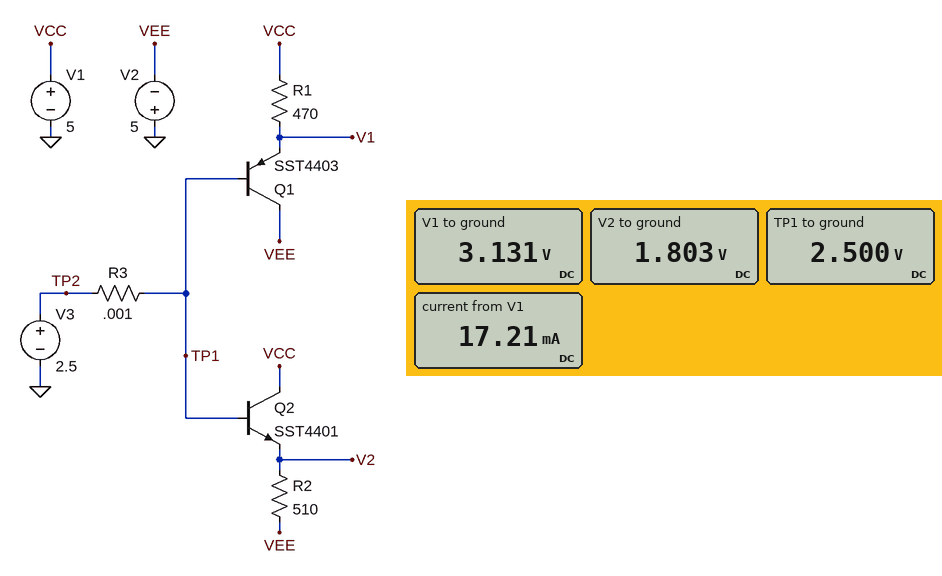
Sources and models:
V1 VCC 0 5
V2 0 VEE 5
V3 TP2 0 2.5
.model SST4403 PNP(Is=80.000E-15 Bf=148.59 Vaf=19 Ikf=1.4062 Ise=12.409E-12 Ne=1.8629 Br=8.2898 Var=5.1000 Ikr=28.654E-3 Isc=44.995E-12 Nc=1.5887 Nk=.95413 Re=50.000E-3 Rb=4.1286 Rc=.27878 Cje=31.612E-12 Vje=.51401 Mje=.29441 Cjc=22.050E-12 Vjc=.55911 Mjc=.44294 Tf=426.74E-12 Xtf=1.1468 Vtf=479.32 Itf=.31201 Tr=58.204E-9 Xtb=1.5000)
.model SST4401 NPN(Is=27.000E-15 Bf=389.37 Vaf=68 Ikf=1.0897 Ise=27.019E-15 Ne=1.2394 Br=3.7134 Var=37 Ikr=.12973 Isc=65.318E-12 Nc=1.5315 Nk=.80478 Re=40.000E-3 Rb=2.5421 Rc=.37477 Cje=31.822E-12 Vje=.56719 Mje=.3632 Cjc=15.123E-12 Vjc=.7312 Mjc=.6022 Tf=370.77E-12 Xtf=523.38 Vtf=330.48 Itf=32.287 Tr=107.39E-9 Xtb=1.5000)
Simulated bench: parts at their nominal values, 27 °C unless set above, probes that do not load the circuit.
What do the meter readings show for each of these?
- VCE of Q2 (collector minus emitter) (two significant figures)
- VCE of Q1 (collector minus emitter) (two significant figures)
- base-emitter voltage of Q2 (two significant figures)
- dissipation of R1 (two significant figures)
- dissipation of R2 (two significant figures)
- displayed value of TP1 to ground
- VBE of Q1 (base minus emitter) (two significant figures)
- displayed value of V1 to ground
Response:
3.2 V
-8.1 V
700 mV
7.4 mW
91 mW
2.500 V
-630 mV
3.131 V
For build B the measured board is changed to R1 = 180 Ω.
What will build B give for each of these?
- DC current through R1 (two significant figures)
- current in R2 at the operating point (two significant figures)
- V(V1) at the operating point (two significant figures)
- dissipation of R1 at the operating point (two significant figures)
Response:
10 mA
13 mA
3.2 V
19 mW
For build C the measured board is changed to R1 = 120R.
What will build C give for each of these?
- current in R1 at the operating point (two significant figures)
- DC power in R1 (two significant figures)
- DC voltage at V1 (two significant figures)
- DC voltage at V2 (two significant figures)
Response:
15 mA
28 mW
3.2 V
1.8 V
